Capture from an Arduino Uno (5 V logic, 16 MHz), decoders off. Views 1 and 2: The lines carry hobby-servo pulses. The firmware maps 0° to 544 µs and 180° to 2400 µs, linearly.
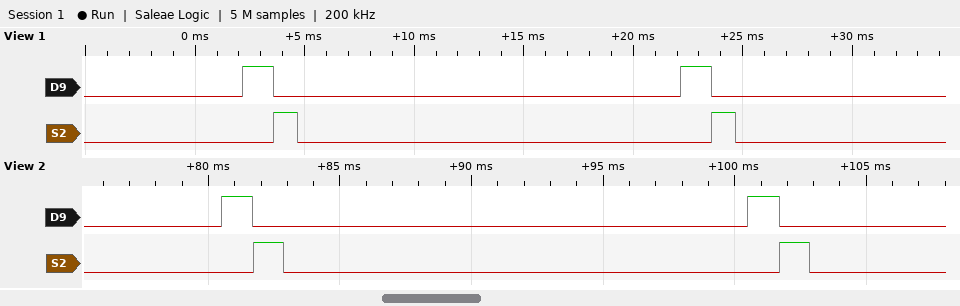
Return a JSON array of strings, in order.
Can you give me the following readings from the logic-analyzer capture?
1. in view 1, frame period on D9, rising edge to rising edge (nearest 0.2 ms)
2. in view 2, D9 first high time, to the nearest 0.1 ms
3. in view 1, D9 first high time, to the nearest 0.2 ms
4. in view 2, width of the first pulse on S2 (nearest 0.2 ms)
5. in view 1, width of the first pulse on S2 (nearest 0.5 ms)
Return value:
["20.0 ms", "1.2 ms", "1.4 ms", "1.2 ms", "1.0 ms"]
